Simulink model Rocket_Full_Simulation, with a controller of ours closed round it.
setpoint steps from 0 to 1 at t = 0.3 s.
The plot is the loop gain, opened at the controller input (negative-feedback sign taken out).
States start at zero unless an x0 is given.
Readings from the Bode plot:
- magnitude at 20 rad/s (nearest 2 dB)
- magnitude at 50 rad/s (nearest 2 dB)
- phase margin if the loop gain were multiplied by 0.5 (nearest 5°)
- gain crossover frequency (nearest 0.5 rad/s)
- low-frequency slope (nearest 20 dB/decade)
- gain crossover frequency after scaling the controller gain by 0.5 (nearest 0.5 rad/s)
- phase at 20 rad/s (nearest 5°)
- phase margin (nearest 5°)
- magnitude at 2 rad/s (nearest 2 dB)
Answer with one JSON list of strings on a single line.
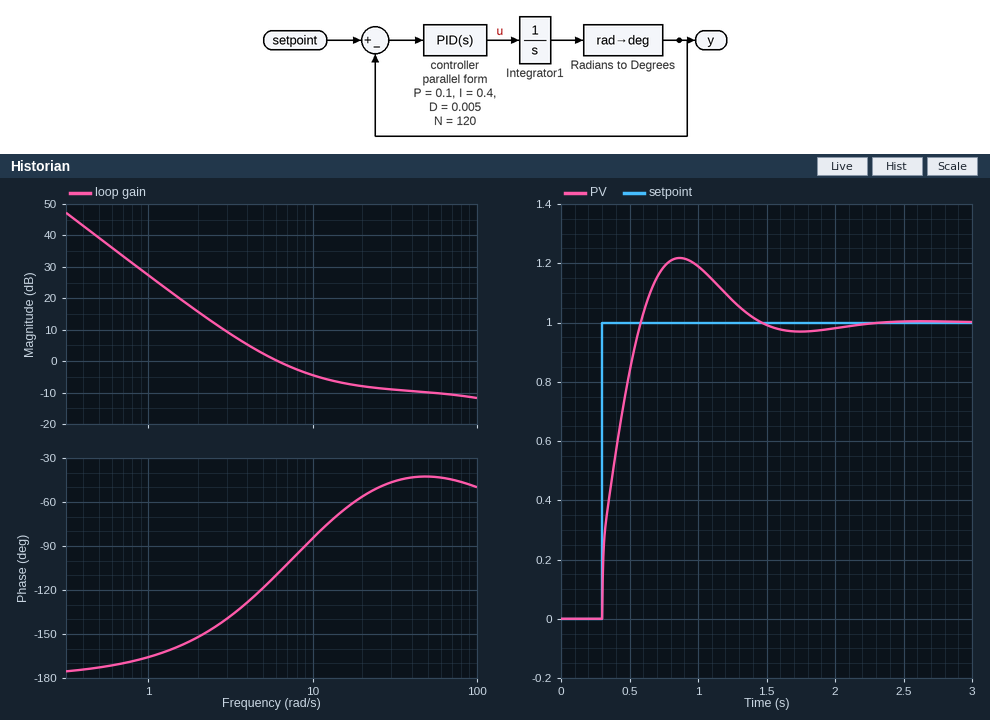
["-8 dB", "-10 dB", "50°", "6.0 rad/s", "-40 dB/decade", "4.0 rad/s", "-55°", "70°", "16 dB"]
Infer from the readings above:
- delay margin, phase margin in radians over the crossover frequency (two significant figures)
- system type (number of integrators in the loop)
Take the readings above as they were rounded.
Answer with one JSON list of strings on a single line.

["0.20 s", "2"]
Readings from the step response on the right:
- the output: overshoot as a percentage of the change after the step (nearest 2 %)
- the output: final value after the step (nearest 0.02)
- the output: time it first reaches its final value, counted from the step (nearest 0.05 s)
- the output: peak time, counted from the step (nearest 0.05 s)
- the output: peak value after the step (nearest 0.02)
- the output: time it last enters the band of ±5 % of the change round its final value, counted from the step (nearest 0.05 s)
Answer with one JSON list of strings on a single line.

["22 %", "1.00", "0.30 s", "0.55 s", "1.22", "1.00 s"]
